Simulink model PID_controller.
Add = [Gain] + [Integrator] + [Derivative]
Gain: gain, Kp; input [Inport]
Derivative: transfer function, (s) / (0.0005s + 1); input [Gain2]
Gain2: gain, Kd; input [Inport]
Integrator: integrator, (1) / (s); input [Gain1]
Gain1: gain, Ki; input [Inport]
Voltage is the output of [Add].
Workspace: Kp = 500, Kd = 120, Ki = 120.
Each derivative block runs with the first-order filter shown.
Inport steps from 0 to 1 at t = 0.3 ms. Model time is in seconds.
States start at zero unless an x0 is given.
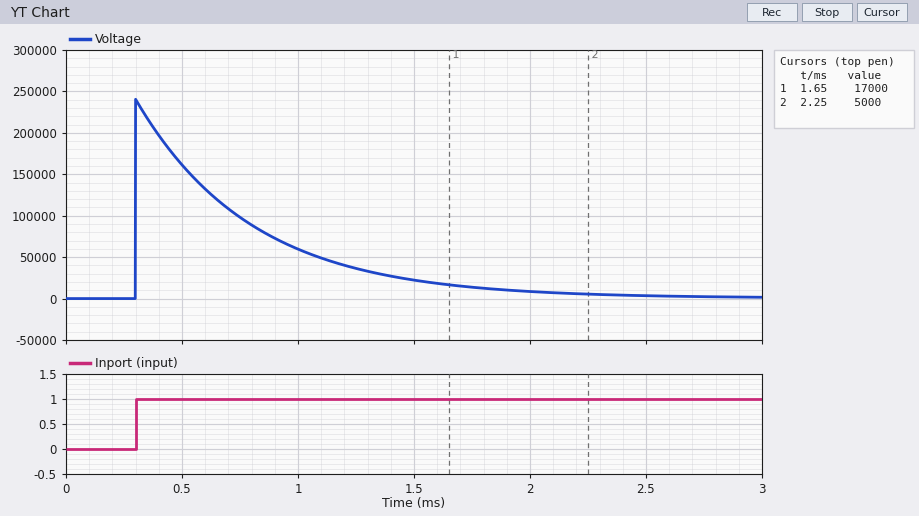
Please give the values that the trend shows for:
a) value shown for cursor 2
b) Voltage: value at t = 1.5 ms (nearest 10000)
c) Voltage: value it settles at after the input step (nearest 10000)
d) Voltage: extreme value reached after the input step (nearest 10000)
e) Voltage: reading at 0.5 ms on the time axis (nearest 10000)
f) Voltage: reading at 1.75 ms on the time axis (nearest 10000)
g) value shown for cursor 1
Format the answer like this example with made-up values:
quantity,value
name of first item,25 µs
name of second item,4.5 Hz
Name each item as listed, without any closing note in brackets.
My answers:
quantity,value
value shown for cursor 2,5000
Voltage: value at t = 1.5 ms,20000
Voltage: value it settles at after the input step,0
Voltage: extreme value reached after the input step,240000
Voltage: reading at 0.5 ms on the time axis,160000
Voltage: reading at 1.75 ms on the time axis,10000
value shown for cursor 1,17000
